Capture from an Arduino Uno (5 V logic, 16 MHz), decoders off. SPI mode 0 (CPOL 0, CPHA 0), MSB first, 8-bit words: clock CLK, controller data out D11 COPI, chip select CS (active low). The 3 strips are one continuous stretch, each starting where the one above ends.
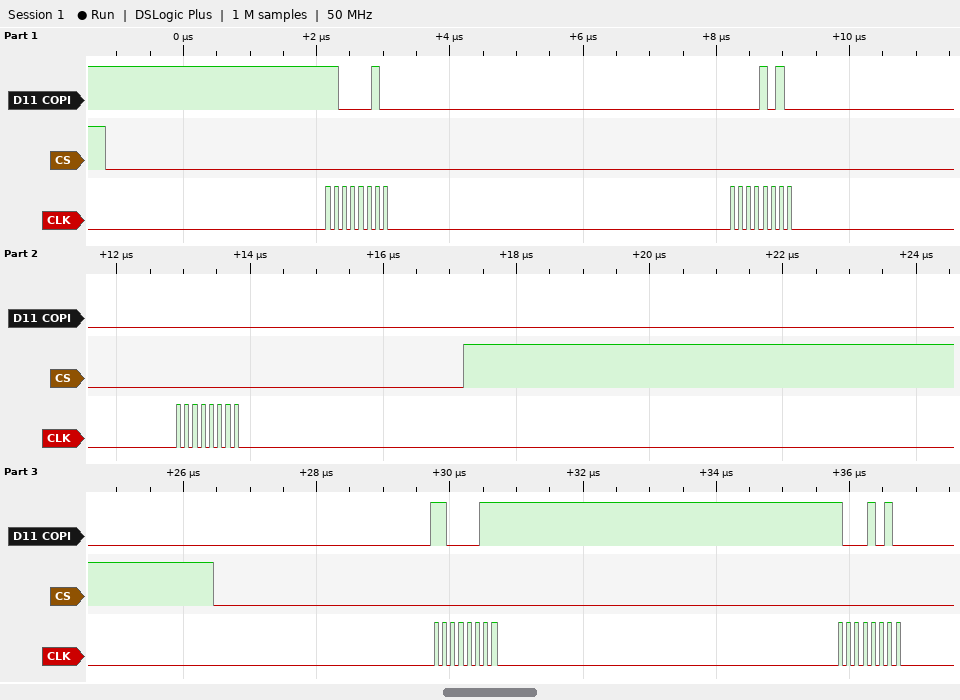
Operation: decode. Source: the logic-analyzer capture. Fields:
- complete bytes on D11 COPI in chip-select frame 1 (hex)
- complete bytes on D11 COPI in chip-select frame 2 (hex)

C2 0A 00
C3 8A
